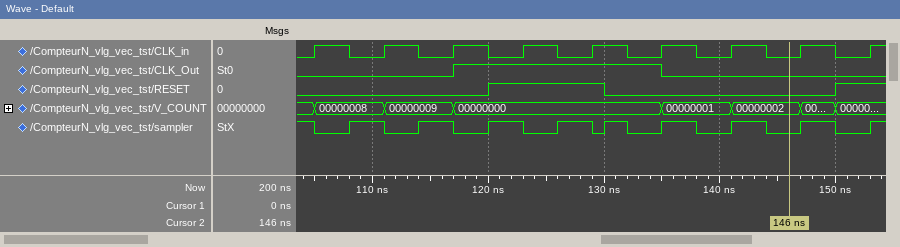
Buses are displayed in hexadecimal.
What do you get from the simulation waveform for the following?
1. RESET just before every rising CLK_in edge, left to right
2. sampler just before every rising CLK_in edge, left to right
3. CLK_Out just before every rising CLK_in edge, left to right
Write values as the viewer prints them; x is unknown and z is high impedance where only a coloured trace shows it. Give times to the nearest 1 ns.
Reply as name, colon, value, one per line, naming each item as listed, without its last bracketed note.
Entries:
RESET just before every rising CLK_in edge, left to right: 0 0 0 1 1 0 0 0 1
sampler just before every rising CLK_in edge, left to right: 1 1 1 1 1 0 0 0 0
CLK_Out just before every rising CLK_in edge, left to right: 0 0 0 1 1 1 0 0 0
